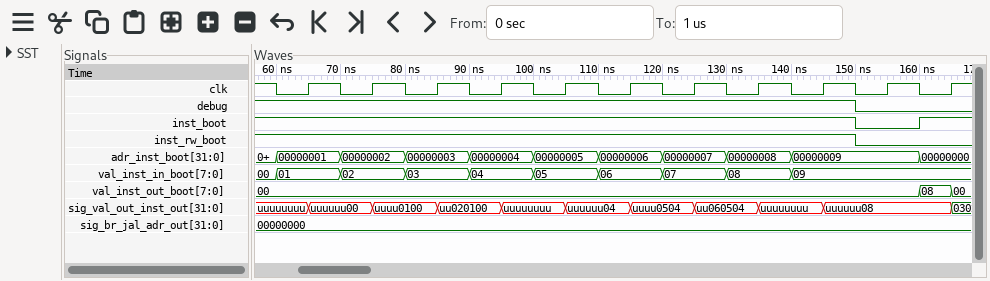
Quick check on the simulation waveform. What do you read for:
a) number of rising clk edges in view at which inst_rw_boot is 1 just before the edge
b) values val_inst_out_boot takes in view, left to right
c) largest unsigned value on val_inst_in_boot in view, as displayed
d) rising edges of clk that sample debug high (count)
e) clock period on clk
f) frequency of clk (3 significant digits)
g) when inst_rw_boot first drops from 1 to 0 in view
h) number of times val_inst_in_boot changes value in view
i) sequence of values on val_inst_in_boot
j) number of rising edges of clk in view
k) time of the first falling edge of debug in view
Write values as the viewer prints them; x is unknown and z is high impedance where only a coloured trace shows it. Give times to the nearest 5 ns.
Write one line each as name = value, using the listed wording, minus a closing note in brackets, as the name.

number of rising clk edges in view at which inst_rw_boot is 1 just before the edge = 9
values val_inst_out_boot takes in view, left to right = 00, 08, 00
largest unsigned value on val_inst_in_boot in view, as displayed = 09
rising edges of clk that sample debug high = 9
clock period on clk = 10 ns
frequency of clk = 100 MHz
when inst_rw_boot first drops from 1 to 0 in view = 150 ns
number of times val_inst_in_boot changes value in view = 9
sequence of values on val_inst_in_boot = 00, 01, 02, 03, 04, 05, 06, 07, 08, 09
number of rising edges of clk in view = 11
time of the first falling edge of debug in view = 150 ns
